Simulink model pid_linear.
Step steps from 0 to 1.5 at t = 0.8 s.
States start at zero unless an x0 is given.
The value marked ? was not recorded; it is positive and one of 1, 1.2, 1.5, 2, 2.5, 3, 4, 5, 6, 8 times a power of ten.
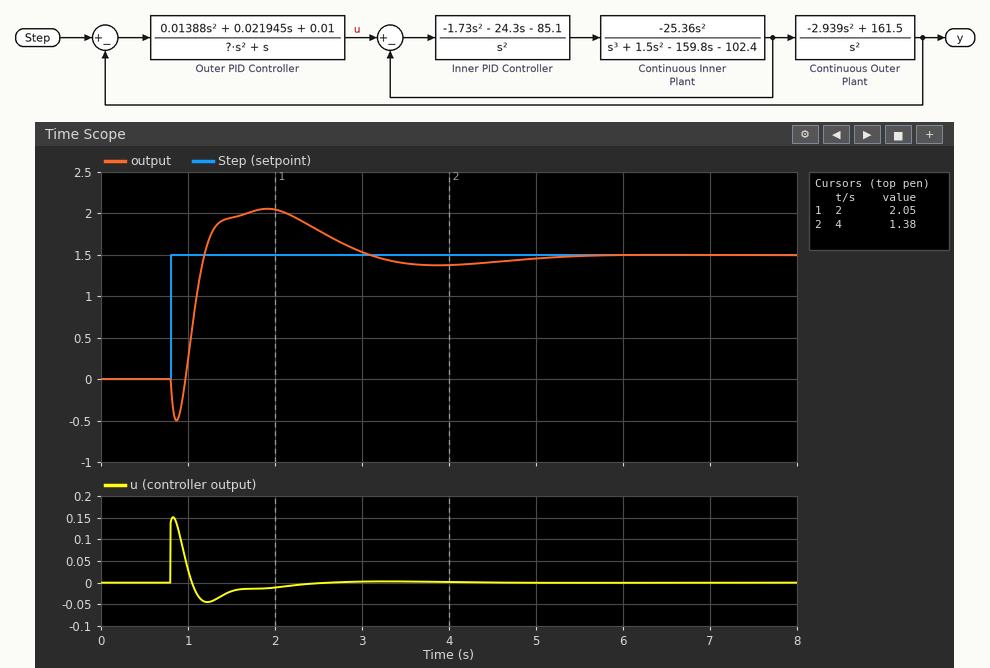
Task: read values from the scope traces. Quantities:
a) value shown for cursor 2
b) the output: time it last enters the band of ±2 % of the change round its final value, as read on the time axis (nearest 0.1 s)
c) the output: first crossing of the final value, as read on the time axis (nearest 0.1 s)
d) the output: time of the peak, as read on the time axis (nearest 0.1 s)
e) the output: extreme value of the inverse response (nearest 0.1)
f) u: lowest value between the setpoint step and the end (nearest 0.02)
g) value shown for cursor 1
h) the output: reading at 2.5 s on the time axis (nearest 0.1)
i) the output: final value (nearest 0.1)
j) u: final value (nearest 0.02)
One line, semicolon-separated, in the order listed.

1.38; 5.2 s; 1.2 s; 1.9 s; -0.5; -0.04; 2.05; 1.8; 1.5; 0.00
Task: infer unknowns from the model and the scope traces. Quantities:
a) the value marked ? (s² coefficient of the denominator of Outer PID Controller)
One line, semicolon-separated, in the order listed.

0.15
